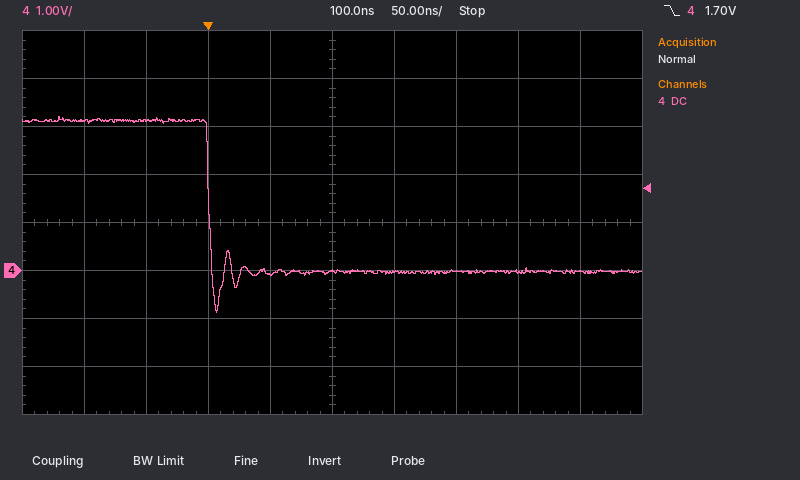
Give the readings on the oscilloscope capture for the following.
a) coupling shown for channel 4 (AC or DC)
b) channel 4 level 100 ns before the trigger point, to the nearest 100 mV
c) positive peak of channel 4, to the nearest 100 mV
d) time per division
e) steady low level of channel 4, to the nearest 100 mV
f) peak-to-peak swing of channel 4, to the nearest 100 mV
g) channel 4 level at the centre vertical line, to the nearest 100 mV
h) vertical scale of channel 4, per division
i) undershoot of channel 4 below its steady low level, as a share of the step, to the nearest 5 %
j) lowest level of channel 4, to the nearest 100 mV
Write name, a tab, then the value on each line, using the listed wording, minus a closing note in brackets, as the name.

coupling shown for channel 4	DC
channel 4 level 100 ns before the trigger point, to the nearest 100 mV	3.1 V
positive peak of channel 4, to the nearest 100 mV	3.2 V
time per division	50 ns
steady low level of channel 4, to the nearest 100 mV	0.0 V
peak-to-peak swing of channel 4, to the nearest 100 mV	4.1 V
channel 4 level at the centre vertical line, to the nearest 100 mV	0.0 V
vertical scale of channel 4, per division	1 V
undershoot of channel 4 below its steady low level, as a share of the step, to the nearest 5 %	25 %
lowest level of channel 4, to the nearest 100 mV	-900 mV
